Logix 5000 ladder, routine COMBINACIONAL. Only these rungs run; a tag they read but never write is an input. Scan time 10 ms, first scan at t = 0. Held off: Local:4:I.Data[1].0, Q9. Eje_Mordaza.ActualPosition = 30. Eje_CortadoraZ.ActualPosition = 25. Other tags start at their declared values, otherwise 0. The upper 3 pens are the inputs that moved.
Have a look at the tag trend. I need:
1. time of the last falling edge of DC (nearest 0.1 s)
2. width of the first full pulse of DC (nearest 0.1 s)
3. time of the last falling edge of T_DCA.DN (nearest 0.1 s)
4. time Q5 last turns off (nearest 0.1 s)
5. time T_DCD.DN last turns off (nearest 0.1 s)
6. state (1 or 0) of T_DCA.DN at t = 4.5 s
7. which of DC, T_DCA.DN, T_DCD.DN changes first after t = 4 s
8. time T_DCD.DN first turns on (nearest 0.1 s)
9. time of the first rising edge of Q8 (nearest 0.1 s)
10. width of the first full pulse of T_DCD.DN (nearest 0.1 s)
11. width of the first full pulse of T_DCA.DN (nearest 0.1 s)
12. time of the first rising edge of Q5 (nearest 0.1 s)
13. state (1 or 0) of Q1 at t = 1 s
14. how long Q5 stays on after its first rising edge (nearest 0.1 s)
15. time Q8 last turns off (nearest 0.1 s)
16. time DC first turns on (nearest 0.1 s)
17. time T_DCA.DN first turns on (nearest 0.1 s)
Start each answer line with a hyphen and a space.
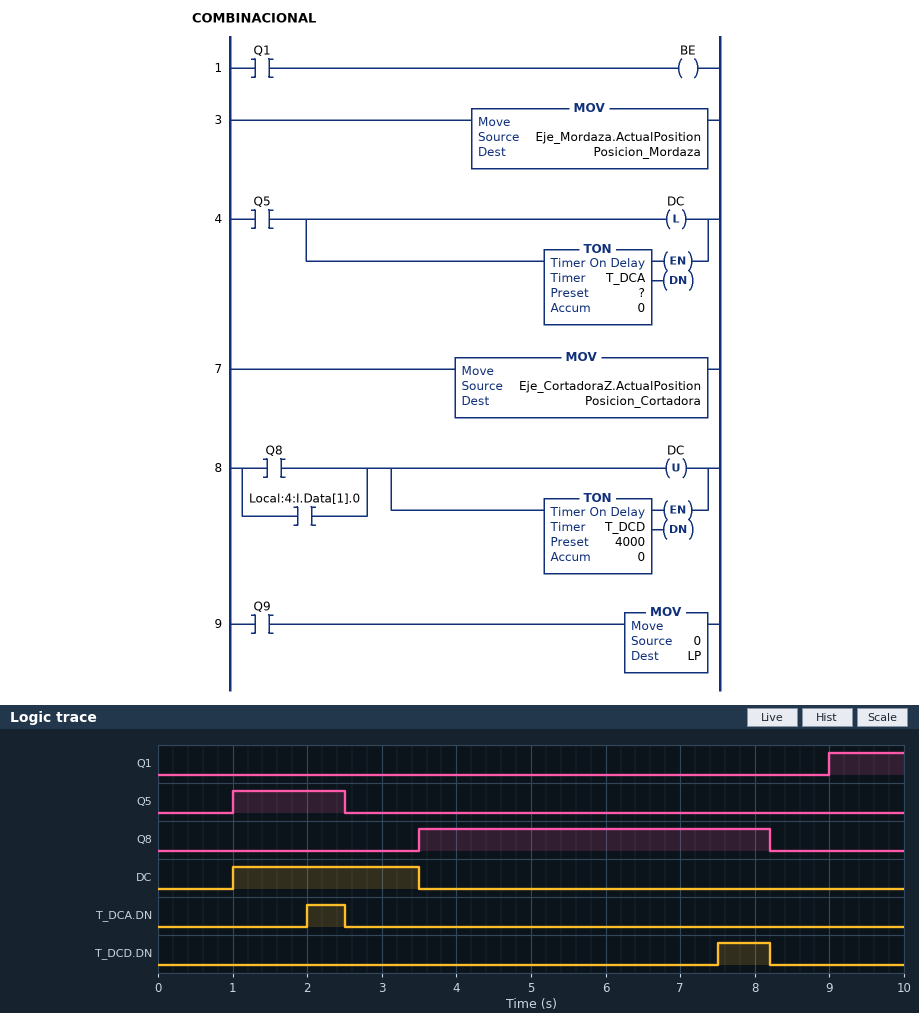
- 3.5 s
- 2.5 s
- 2.5 s
- 2.5 s
- 8.2 s
- 0
- T_DCD.DN
- 7.5 s
- 3.5 s
- 0.7 s
- 0.5 s
- 1.0 s
- 0
- 1.5 s
- 8.2 s
- 1.0 s
- 2.0 s
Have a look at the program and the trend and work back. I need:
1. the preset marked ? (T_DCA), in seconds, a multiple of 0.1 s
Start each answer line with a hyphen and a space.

- 1.0 s
